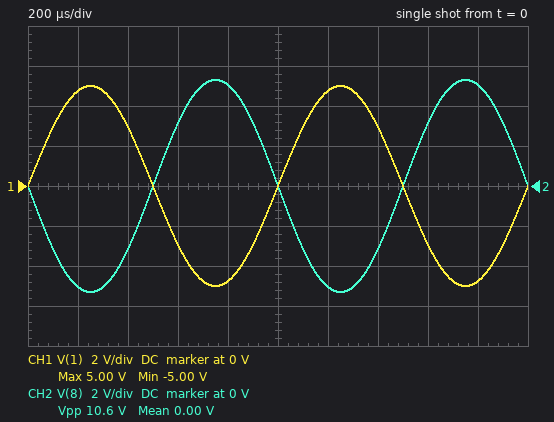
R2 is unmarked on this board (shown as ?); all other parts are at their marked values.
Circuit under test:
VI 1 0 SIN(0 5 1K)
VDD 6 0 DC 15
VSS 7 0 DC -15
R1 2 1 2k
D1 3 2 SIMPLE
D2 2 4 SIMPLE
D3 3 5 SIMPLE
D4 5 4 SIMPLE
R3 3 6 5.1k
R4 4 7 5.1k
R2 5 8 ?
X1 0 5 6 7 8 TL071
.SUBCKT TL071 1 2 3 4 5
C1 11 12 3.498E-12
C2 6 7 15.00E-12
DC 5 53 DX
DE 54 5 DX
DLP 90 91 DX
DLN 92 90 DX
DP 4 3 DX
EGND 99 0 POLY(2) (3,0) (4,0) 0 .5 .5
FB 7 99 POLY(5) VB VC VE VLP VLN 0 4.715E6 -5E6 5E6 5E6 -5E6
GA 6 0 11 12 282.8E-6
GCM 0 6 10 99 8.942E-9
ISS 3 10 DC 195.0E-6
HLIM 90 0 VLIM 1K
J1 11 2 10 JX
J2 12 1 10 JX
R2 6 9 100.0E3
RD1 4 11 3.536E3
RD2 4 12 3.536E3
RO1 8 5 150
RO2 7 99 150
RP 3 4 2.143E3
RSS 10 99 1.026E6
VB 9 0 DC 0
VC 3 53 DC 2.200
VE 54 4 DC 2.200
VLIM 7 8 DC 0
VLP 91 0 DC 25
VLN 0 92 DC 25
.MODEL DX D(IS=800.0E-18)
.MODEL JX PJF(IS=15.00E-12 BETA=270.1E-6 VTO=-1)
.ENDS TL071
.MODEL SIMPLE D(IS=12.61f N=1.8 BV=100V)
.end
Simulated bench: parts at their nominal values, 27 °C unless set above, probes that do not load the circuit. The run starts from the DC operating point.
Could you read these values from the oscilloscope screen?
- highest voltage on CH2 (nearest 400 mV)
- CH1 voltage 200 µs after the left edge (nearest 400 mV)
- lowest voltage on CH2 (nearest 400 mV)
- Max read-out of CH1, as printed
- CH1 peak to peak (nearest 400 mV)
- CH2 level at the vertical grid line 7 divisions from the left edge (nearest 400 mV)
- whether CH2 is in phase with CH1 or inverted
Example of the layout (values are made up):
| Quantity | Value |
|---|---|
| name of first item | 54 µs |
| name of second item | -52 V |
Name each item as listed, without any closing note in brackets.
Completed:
| Quantity | Value |
|---|---|
| highest voltage on CH2 | 5.2 V |
| CH1 voltage 200 µs after the left edge | 4.8 V |
| lowest voltage on CH2 | -5.2 V |
| Max read-out of CH1, as printed | 5.00 V |
| CH1 peak to peak | 10.0 V |
| CH2 level at the vertical grid line 7 divisions from the left edge | -3.2 V |
| whether CH2 is in phase with CH1 or inverted | inverted |
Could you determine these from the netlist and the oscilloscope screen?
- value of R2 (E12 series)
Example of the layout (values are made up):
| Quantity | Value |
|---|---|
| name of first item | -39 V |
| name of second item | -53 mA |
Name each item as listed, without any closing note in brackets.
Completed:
| Quantity | Value |
|---|---|
| value of R2 | 2.2 kΩ |
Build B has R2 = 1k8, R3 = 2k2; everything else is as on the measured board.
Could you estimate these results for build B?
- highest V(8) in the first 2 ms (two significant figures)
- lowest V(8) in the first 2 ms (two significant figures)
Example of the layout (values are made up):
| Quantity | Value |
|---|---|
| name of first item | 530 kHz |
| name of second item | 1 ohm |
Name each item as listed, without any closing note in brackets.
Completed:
| Quantity | Value |
|---|---|
| highest V(8) in the first 2 ms | -1.9 V |
| lowest V(8) in the first 2 ms | -11 V |
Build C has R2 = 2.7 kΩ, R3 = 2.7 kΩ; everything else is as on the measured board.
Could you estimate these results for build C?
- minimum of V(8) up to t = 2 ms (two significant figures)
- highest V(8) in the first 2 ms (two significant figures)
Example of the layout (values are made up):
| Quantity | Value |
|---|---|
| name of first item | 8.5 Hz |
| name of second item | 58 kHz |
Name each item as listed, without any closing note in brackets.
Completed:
| Quantity | Value |
|---|---|
| minimum of V(8) up to t = 2 ms | -13 V |
| highest V(8) in the first 2 ms | 210 mV |
